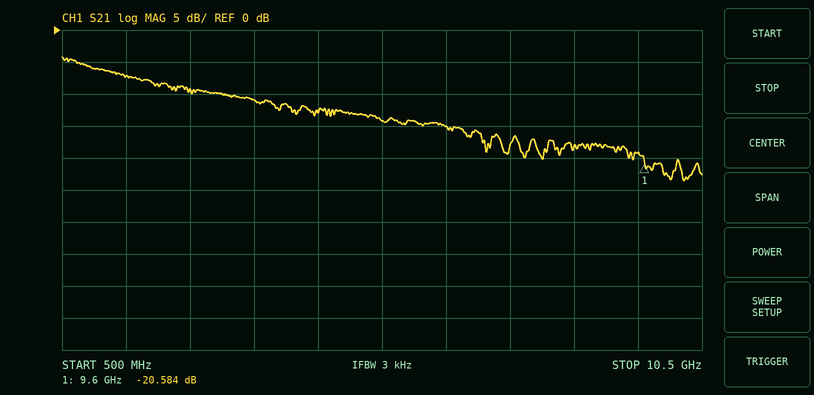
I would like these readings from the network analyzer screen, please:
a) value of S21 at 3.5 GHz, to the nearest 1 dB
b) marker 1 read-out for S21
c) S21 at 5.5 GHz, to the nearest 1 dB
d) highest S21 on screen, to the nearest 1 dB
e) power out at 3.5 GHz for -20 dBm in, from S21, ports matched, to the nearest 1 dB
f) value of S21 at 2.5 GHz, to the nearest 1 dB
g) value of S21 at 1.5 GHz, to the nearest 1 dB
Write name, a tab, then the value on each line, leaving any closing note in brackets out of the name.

value of S21 at 3.5 GHz, to the nearest 1 dB	-11 dB
marker 1 read-out for S21	-20.584 dB
S21 at 5.5 GHz, to the nearest 1 dB	-14 dB
highest S21 on screen, to the nearest 1 dB	-4 dB
power out at 3.5 GHz for -20 dBm in, from S21, ports matched, to the nearest 1 dB	-31 dBm
value of S21 at 2.5 GHz, to the nearest 1 dB	-9 dB
value of S21 at 1.5 GHz, to the nearest 1 dB	-7 dB
